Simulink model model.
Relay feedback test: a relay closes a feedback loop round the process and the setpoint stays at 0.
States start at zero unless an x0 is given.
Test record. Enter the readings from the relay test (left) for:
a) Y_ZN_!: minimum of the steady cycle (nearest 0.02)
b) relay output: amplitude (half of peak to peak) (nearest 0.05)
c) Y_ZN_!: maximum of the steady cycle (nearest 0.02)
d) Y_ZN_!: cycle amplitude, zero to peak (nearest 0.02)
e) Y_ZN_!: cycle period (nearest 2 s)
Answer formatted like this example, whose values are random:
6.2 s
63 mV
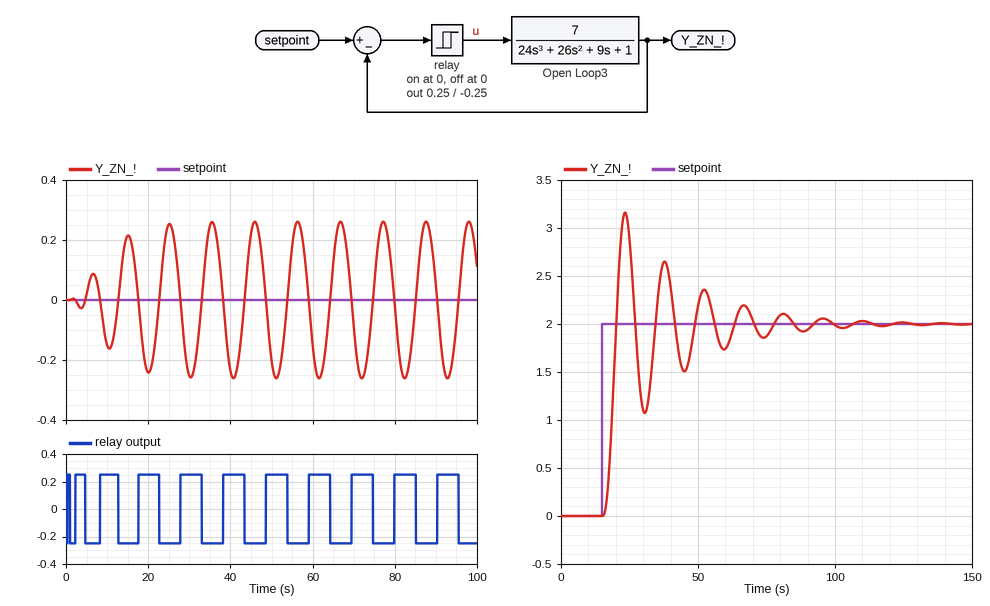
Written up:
-0.26
0.25
0.26
0.26
10 s
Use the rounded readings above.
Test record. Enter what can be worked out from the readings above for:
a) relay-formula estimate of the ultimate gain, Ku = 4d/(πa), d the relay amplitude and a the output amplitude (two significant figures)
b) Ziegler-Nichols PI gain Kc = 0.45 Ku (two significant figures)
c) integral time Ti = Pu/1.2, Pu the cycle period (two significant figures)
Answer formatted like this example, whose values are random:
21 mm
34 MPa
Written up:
1.2
0.54
8.3 s
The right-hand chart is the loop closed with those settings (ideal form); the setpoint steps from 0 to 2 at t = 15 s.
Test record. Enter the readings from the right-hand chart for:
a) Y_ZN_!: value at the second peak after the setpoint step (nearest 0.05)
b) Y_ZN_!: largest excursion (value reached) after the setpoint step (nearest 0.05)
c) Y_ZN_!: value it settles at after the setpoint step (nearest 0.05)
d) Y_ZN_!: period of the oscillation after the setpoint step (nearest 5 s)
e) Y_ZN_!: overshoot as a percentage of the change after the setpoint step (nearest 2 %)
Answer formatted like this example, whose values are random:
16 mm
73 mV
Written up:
2.65
3.15
2.00
15 s
58 %
